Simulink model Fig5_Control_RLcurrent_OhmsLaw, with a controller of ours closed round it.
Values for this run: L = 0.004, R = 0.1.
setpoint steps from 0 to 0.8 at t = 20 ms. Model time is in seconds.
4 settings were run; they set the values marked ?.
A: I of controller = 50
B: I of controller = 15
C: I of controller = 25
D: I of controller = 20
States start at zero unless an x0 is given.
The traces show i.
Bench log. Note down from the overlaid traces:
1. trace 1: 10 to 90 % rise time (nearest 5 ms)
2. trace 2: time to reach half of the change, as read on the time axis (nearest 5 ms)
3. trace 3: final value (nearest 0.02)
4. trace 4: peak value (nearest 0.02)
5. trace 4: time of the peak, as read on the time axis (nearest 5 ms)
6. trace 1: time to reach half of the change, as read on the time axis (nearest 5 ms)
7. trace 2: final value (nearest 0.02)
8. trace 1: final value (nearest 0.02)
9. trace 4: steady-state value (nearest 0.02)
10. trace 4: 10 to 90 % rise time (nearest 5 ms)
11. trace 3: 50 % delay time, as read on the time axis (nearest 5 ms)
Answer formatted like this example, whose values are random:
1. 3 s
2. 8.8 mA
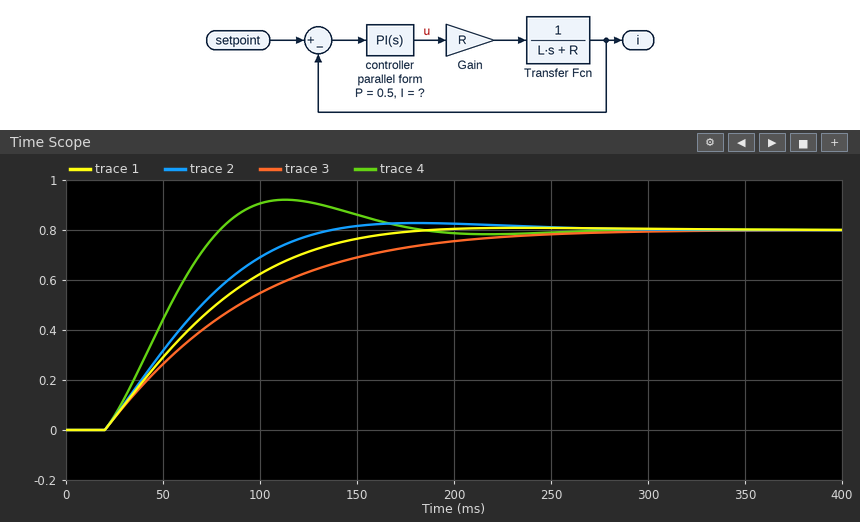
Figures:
1. 100 ms
2. 60 ms
3. 0.80
4. 0.92
5. 115 ms
6. 65 ms
7. 0.80
8. 0.80
9. 0.80
10. 45 ms
11. 70 ms
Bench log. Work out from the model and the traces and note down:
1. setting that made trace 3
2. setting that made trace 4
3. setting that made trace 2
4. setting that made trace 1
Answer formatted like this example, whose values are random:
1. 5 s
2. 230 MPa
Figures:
1. B
2. A
3. C
4. D
